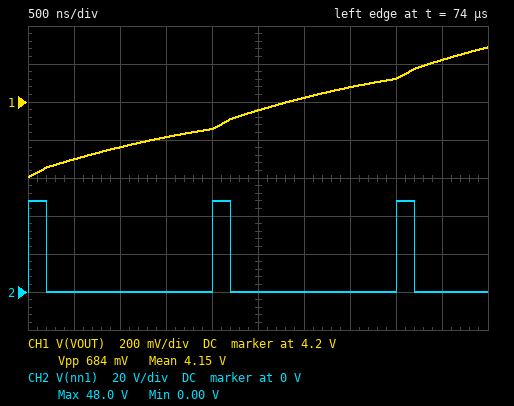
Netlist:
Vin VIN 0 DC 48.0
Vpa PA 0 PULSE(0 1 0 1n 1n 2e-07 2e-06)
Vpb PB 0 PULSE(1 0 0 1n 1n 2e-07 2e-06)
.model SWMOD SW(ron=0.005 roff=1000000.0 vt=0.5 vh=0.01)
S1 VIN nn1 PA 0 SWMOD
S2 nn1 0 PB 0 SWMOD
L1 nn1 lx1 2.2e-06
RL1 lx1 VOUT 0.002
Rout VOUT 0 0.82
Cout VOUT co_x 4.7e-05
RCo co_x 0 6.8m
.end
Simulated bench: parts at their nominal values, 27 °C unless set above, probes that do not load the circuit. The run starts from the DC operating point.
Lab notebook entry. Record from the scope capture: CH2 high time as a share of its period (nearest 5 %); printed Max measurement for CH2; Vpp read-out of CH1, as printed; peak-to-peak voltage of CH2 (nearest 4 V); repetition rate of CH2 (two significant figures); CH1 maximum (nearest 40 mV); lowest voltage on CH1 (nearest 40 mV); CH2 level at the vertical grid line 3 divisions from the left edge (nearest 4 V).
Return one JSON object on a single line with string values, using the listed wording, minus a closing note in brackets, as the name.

{"CH2 high time as a share of its period": "10 %", "printed Max measurement for CH2": "48.0 V", "Vpp read-out of CH1, as printed": "684 mV", "peak-to-peak voltage of CH2": "48 V", "repetition rate of CH2": "500 kHz", "CH1 maximum": "4.48 V", "lowest voltage on CH1": "3.80 V", "CH2 level at the vertical grid line 3 divisions from the left edge": "0 V"}
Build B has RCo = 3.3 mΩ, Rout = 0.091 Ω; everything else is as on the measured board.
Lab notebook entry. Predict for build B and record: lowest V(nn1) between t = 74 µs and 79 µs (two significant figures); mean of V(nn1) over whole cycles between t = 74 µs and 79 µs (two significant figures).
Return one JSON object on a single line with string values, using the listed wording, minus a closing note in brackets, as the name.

{"lowest V(nn1) between t = 74 µs and 79 µs": "-250 mV", "mean of V(nn1) over whole cycles between t = 74 µs and 79 µs": "4.6 V"}
